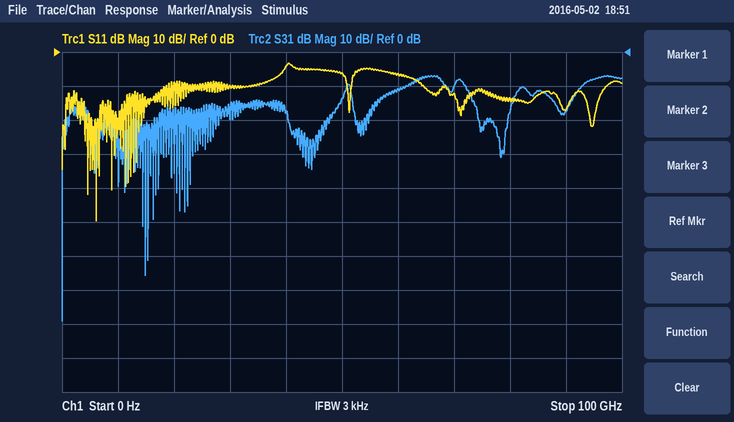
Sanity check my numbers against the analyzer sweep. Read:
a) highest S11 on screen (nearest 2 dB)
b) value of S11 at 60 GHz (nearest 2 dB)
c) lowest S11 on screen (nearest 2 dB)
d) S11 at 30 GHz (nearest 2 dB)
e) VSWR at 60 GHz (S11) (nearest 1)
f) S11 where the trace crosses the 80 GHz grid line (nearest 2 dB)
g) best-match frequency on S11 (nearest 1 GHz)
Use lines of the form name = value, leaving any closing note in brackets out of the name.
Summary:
highest S11 on screen = -4 dB
value of S11 at 60 GHz = -6 dB
lowest S11 on screen = -50 dB
S11 at 30 GHz = -10 dB
VSWR at 60 GHz (S11) = 3
S11 where the trace crosses the 80 GHz grid line = -14 dB
best-match frequency on S11 = 6 GHz
